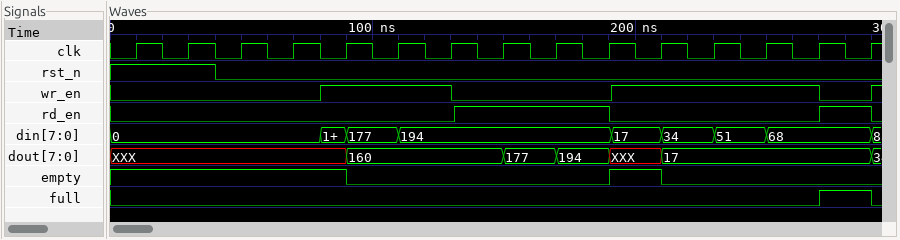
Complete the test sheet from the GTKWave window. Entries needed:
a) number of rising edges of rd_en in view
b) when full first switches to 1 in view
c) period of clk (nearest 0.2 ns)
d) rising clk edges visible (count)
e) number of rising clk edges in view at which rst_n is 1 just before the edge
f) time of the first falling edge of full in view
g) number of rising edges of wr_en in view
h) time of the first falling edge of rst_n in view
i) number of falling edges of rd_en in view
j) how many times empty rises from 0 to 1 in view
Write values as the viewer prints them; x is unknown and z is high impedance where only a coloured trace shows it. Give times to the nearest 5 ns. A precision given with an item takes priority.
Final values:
2
270 ns
20 ns
15
2
290 ns
3
40 ns
2
1
